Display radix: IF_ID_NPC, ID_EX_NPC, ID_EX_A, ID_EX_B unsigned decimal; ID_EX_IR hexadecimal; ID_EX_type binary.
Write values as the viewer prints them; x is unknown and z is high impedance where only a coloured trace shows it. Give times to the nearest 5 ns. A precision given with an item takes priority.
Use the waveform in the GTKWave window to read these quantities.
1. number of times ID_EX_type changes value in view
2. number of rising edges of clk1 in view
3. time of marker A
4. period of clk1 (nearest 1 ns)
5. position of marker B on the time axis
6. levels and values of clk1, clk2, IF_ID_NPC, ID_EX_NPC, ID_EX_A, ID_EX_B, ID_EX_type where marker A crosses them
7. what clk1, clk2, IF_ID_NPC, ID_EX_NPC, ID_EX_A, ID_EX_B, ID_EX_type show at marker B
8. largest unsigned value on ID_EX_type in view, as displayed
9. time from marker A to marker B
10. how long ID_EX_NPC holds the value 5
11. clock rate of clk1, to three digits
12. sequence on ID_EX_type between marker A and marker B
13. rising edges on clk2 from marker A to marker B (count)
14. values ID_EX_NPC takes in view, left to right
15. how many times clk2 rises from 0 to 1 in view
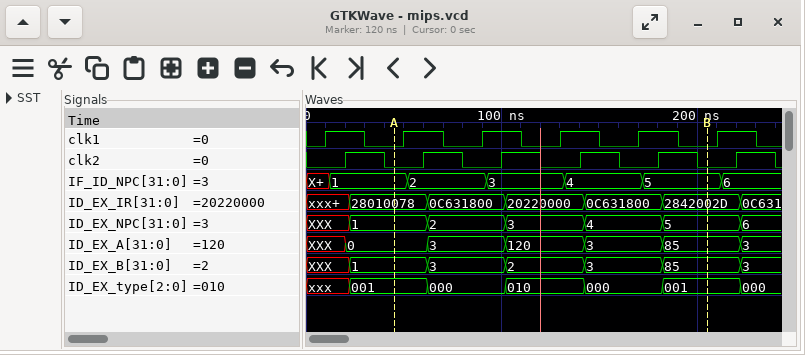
6
6
45 ns
40 ns
205 ns
clk1=0, clk2=0, IF_ID_NPC=1, ID_EX_NPC=1, ID_EX_A=0, ID_EX_B=1, ID_EX_type=001
clk1=0, clk2=0, IF_ID_NPC=5, ID_EX_NPC=5, ID_EX_A=85, ID_EX_B=85, ID_EX_type=001
010
160 ns
40 ns
25.0 MHz
001, 000, 010, 000, 001
4
XXX, 1, 2, 3, 4, 5, 6
6
